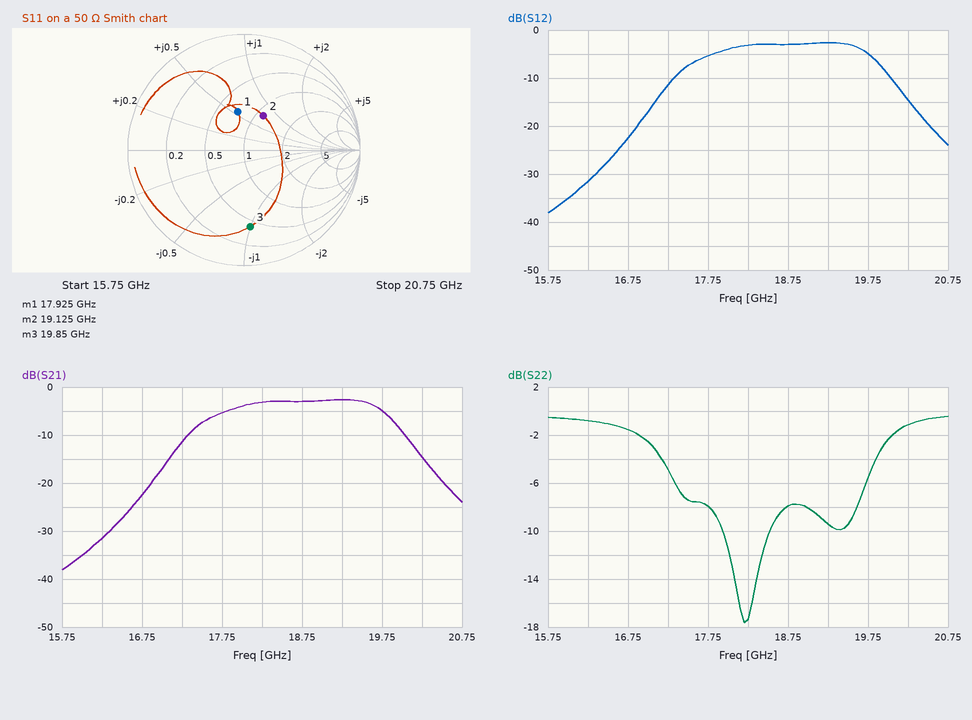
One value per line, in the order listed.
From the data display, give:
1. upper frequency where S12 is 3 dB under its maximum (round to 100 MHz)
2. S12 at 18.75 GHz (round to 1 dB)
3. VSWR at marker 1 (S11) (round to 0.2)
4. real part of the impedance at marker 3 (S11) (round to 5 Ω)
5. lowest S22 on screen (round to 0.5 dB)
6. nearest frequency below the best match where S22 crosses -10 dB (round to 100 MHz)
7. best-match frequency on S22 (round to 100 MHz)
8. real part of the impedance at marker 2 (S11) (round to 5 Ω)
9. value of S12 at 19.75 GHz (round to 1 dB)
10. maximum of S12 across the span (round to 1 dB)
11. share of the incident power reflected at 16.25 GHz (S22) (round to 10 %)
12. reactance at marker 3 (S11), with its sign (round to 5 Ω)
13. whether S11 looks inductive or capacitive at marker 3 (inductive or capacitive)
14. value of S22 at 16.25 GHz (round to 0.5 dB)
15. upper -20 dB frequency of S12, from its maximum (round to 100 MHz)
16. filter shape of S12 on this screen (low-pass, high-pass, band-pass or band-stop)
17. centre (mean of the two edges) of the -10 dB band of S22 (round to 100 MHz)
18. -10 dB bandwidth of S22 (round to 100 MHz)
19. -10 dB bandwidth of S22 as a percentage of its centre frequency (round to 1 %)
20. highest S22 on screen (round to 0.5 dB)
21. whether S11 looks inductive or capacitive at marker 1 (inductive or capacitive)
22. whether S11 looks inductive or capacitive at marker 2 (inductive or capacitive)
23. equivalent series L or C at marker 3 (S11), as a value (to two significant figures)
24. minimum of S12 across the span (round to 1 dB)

19.8 GHz
-3 dB
2.0
20 Ω
-17.5 dB
17.9 GHz
18.2 GHz
55 Ω
-5 dB
-3 dB
80 %
-50 Ω
capacitive
-1.0 dB
20.7 GHz
band-pass
18.2 GHz
600 MHz
3 %
-0.5 dB
inductive
inductive
160 fF
-38 dB
